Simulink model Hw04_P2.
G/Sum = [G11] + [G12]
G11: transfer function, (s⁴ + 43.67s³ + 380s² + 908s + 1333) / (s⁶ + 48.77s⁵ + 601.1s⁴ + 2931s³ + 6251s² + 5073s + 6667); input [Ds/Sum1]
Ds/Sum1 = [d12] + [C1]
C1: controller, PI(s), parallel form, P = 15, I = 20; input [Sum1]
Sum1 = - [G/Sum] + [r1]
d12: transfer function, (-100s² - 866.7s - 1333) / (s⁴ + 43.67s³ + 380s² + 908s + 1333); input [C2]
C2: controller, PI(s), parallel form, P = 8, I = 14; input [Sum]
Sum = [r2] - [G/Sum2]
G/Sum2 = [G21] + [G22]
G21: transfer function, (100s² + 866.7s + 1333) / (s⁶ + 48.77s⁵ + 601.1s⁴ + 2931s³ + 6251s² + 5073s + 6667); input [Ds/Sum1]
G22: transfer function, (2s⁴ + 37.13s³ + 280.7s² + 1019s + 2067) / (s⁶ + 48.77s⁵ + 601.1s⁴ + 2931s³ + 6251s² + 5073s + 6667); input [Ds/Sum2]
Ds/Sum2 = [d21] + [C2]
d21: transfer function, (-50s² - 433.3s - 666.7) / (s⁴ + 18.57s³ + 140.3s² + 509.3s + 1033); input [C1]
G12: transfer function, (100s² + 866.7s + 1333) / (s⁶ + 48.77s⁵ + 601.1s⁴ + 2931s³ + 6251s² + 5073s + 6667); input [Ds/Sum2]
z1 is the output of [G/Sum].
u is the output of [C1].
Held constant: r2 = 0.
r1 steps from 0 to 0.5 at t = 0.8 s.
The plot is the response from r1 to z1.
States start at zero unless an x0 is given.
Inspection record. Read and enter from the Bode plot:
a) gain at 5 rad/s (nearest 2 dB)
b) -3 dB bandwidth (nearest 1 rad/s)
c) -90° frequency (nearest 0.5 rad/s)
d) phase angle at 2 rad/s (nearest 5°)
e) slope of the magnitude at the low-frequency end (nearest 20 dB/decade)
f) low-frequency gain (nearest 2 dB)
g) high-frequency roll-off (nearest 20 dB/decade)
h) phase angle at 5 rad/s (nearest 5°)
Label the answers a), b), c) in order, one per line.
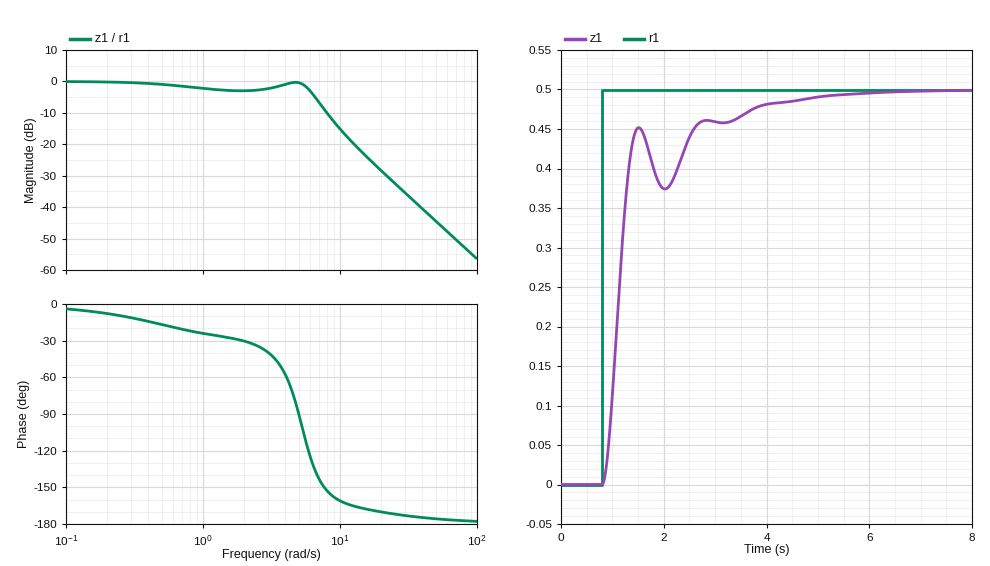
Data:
a) 0 dB
b) 6 rad/s
c) 5.0 rad/s
d) -30°
e) 0 dB/decade
f) 0 dB
g) -40 dB/decade
h) -90°
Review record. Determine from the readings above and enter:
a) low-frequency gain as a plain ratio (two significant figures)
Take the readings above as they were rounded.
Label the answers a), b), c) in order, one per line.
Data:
a) 1.0
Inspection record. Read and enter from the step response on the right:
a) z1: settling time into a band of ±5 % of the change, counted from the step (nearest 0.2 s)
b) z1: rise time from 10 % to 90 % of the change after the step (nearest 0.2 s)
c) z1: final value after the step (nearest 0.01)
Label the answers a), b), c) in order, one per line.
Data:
a) 3.0 s
b) 0.6 s
c) 0.50
